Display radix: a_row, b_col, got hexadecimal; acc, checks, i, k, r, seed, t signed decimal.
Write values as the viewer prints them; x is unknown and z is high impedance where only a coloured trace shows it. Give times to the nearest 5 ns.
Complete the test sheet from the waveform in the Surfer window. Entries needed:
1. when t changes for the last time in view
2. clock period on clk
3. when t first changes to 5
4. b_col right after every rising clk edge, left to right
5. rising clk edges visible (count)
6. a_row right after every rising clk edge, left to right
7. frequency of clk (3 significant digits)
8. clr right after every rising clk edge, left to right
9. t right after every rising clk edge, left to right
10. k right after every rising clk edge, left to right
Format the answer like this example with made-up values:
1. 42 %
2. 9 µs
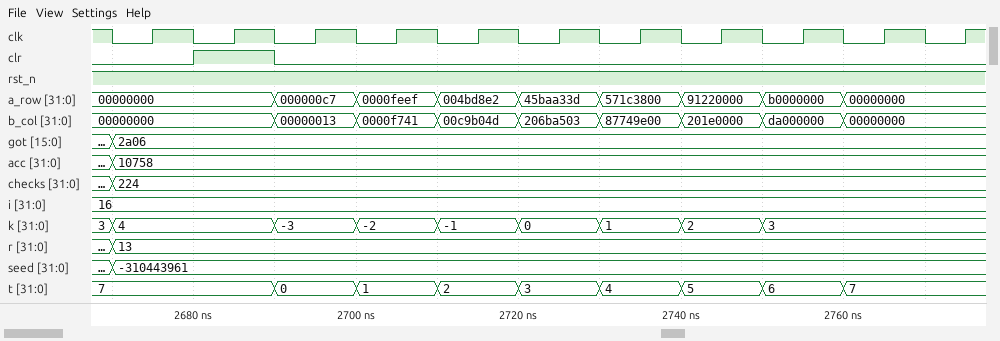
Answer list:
1. 2760 ns
2. 10 ns
3. 2740 ns
4. 00000000, 00000000, 00000013, 0000f741, 00c9b04d, 206ba503, 87749e00, 201e0000, da000000, 00000000, 00000000
5. 11
6. 00000000, 00000000, 000000c7, 0000feef, 004bd8e2, 45baa33d, 571c3800, 91220000, b0000000, 00000000, 00000000
7. 100 MHz
8. 0 1 0 0 0 0 0 0 0 0 0
9. 7, 7, 0, 1, 2, 3, 4, 5, 6, 7, 7
10. 4, 4, -3, -2, -1, 0, 1, 2, 3, 3, 3
